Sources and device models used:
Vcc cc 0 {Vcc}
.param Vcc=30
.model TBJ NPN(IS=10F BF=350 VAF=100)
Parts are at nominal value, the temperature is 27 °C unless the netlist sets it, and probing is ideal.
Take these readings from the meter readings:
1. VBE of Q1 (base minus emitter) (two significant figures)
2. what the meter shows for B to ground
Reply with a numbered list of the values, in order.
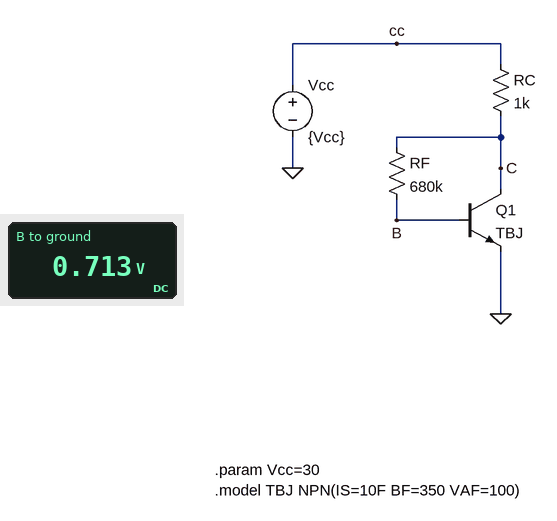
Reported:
1. 710 mV
2. 0.713 V
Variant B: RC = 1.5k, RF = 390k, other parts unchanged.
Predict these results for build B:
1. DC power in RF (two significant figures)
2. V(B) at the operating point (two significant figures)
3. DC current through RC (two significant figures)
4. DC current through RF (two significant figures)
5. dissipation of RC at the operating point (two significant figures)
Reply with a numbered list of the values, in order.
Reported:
1. 350 µW
2. 720 mV
3. 12 mA
4. 30 µA
5. 210 mW
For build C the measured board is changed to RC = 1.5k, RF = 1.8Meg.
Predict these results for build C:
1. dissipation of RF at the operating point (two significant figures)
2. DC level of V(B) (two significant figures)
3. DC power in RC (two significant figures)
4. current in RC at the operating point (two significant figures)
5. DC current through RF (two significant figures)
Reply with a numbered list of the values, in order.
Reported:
1. 260 µW
2. 690 mV
3. 39 mW
4. 5.1 mA
5. 12 µA
